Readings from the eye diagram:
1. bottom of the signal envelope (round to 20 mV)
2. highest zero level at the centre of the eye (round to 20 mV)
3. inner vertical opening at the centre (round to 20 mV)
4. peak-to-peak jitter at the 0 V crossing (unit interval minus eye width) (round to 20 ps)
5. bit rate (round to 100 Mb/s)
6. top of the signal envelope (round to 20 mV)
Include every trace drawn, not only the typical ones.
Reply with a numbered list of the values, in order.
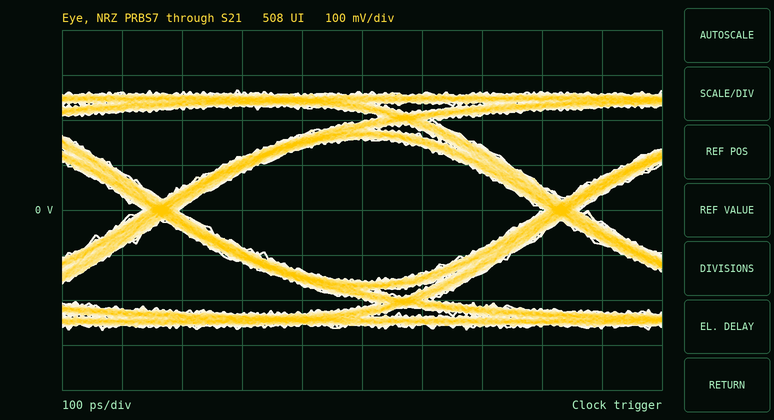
1. -260 mV
2. -160 mV
3. 320 mV
4. 60 ps
5. 1.5 Gb/s
6. 260 mV
